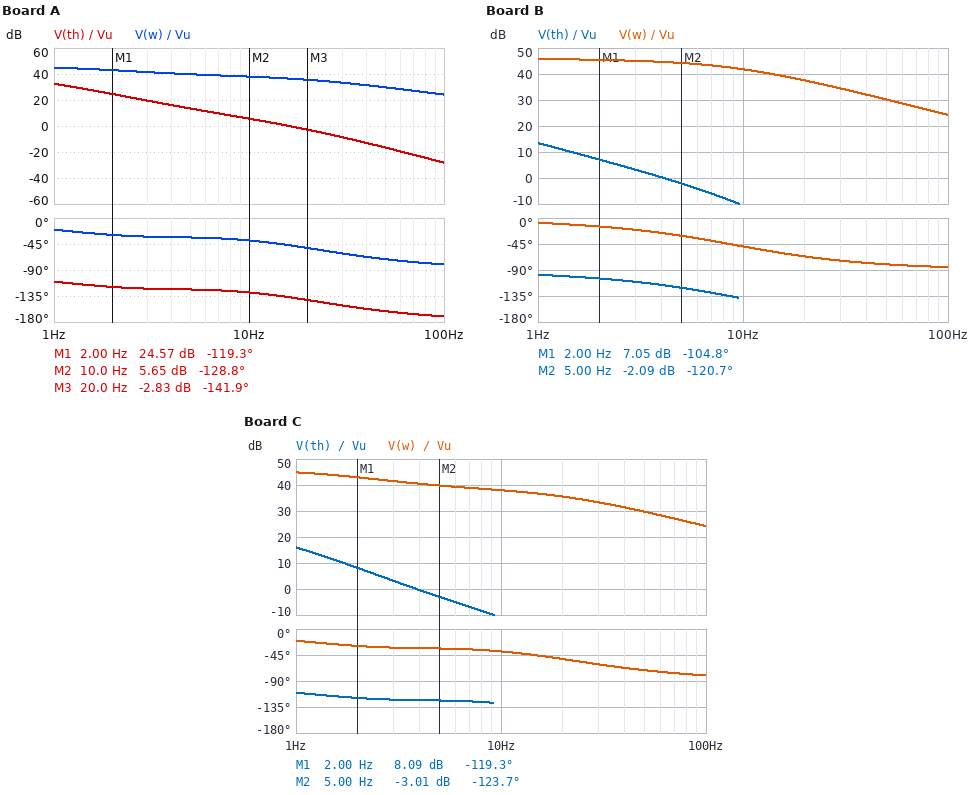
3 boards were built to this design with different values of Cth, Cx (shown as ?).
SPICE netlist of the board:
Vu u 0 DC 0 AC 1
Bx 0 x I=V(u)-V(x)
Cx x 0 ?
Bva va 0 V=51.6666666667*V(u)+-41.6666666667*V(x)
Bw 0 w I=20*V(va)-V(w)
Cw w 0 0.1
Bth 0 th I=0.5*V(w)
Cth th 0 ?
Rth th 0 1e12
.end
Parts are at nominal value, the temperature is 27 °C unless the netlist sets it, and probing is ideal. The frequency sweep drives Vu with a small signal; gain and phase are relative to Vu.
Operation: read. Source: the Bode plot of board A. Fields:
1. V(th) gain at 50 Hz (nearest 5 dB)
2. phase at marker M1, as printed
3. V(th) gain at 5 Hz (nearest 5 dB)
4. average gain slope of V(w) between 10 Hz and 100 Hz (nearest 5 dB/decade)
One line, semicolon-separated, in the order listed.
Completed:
-15 dB; -119.3 deg; 15 dB; -15 dB/decade
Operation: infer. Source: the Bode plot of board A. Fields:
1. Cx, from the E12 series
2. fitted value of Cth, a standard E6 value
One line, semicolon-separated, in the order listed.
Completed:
8.2 mF; 330 mF
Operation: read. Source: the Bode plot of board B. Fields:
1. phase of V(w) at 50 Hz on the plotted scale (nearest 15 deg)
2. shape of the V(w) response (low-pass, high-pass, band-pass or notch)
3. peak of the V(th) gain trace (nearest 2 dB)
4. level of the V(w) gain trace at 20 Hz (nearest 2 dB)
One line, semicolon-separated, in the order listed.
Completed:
-75 deg; low-pass; 14 dB; 38 dB
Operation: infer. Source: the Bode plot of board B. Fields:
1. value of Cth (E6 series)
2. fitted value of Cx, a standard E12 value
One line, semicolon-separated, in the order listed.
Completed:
3.3 F; 18 mF
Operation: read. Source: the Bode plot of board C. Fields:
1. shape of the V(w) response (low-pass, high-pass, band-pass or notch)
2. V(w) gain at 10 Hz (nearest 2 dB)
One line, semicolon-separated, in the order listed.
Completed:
low-pass; 38 dB
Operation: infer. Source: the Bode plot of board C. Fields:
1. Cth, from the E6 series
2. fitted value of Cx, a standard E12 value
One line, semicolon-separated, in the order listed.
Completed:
2.2 F; 8.2 mF
